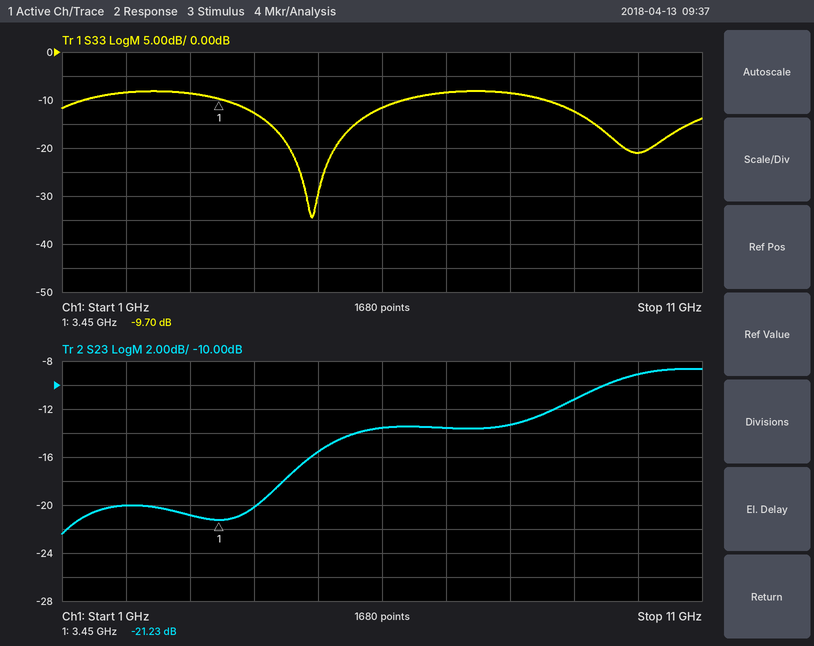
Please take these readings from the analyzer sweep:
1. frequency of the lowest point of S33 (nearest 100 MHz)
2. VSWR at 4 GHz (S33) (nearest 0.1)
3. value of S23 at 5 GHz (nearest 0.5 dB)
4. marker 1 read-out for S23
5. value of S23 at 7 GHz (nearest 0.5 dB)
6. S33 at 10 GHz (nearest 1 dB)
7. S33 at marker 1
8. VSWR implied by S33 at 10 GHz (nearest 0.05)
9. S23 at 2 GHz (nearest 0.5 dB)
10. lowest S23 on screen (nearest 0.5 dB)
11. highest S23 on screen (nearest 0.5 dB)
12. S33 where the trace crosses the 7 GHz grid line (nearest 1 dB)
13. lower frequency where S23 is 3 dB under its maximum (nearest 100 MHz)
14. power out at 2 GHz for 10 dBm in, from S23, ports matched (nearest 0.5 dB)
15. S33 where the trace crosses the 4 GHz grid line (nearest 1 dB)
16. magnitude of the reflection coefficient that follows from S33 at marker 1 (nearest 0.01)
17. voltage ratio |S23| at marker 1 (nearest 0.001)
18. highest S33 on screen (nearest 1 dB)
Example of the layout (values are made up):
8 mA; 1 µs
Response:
4.9 GHz; 1.6; -15.5 dB; -21.23 dB; -13.5 dB; -21 dB; -9.70 dB; 1.20; -20.0 dB; -22.5 dB; -8.5 dB; -8 dB; 8.8 GHz; -10.0 dBm; -13 dB; 0.33; 0.087; -8 dB
